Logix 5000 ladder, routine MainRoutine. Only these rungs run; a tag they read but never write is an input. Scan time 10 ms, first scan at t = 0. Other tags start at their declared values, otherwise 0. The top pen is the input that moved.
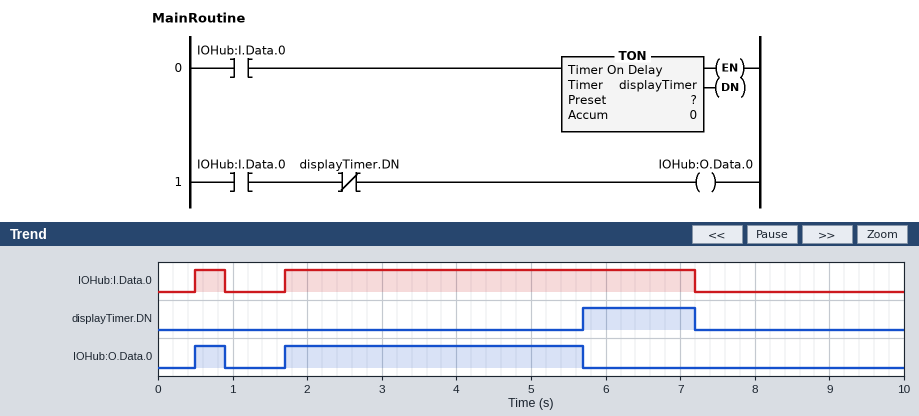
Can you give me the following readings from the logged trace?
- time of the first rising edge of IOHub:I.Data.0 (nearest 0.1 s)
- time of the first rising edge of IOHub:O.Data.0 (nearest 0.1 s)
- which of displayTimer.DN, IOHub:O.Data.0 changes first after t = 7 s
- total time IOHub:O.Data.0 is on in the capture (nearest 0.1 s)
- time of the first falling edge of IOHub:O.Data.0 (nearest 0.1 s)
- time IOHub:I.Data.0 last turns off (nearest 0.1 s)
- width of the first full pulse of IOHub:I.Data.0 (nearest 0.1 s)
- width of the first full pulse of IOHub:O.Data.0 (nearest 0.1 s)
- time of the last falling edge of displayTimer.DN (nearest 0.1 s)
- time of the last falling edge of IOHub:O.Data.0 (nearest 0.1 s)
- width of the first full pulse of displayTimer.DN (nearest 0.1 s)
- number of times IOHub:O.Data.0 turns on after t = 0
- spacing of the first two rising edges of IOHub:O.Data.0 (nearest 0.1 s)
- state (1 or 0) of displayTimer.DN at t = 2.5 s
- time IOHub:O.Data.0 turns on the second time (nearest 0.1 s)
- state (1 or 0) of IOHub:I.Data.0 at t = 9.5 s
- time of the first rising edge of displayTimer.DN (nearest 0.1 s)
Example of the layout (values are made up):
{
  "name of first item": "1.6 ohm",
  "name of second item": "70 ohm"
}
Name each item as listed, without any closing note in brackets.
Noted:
{
  "time of the first rising edge of IOHub:I.Data.0": "0.5 s",
  "time of the first rising edge of IOHub:O.Data.0": "0.5 s",
  "which of displayTimer.DN, IOHub:O.Data.0 changes first after t = 7 s": "displayTimer.DN",
  "total time IOHub:O.Data.0 is on in the capture": "4.4 s",
  "time of the first falling edge of IOHub:O.Data.0": "0.9 s",
  "time IOHub:I.Data.0 last turns off": "7.2 s",
  "width of the first full pulse of IOHub:I.Data.0": "0.4 s",
  "width of the first full pulse of IOHub:O.Data.0": "0.4 s",
  "time of the last falling edge of displayTimer.DN": "7.2 s",
  "time of the last falling edge of IOHub:O.Data.0": "5.7 s",
  "width of the first full pulse of displayTimer.DN": "1.5 s",
  "number of times IOHub:O.Data.0 turns on after t = 0": "2",
  "spacing of the first two rising edges of IOHub:O.Data.0": "1.2 s",
  "state (1 or 0) of displayTimer.DN at t = 2.5 s": "0",
  "time IOHub:O.Data.0 turns on the second time": "1.7 s",
  "state (1 or 0) of IOHub:I.Data.0 at t = 9.5 s": "0",
  "time of the first rising edge of displayTimer.DN": "5.7 s"
}
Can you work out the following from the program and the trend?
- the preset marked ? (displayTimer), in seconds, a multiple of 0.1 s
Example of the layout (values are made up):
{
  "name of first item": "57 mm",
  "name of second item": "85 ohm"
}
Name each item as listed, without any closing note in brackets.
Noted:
{
  "the preset marked ? (displayTimer), in seconds, a multiple of 0.1 s": "4.0 s"
}
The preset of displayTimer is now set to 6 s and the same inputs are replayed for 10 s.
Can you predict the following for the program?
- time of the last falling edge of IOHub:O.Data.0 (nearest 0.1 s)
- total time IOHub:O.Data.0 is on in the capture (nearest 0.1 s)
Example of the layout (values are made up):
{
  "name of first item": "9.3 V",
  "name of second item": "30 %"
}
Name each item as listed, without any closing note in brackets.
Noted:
{
  "time of the last falling edge of IOHub:O.Data.0": "7.2 s",
  "total time IOHub:O.Data.0 is on in the capture": "5.9 s"
}
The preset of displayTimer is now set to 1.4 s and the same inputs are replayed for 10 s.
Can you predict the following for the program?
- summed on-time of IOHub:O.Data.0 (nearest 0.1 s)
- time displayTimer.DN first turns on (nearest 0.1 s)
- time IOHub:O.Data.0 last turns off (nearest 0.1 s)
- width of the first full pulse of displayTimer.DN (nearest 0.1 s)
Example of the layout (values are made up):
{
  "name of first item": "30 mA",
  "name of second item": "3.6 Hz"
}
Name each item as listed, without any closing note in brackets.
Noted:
{
  "summed on-time of IOHub:O.Data.0": "1.8 s",
  "time displayTimer.DN first turns on": "3.1 s",
  "time IOHub:O.Data.0 last turns off": "3.1 s",
  "width of the first full pulse of displayTimer.DN": "4.1 s"
}
